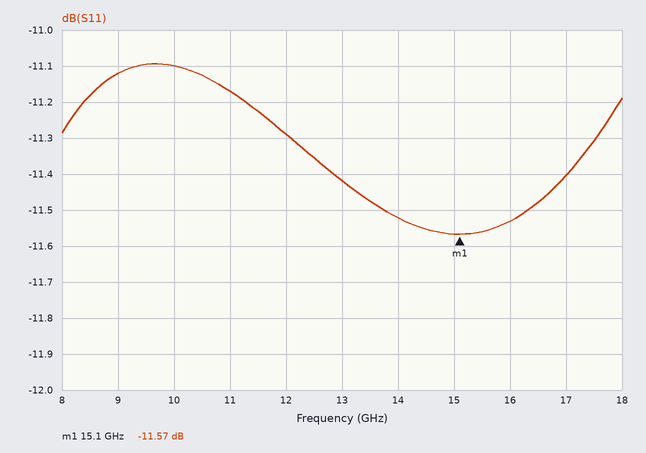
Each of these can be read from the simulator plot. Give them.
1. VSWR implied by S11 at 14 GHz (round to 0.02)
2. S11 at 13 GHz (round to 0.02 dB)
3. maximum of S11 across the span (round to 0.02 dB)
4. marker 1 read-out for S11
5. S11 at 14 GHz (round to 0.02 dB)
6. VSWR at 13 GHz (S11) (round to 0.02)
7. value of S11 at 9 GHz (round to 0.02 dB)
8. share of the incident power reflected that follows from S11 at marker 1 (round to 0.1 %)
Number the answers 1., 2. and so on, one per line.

1. 1.72
2. -11.42 dB
3. -11.10 dB
4. -11.57 dB
5. -11.52 dB
6. 1.74
7. -11.12 dB
8. 7.0 %
